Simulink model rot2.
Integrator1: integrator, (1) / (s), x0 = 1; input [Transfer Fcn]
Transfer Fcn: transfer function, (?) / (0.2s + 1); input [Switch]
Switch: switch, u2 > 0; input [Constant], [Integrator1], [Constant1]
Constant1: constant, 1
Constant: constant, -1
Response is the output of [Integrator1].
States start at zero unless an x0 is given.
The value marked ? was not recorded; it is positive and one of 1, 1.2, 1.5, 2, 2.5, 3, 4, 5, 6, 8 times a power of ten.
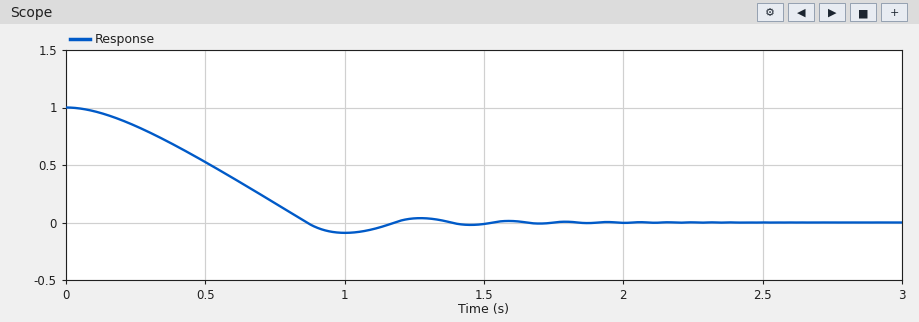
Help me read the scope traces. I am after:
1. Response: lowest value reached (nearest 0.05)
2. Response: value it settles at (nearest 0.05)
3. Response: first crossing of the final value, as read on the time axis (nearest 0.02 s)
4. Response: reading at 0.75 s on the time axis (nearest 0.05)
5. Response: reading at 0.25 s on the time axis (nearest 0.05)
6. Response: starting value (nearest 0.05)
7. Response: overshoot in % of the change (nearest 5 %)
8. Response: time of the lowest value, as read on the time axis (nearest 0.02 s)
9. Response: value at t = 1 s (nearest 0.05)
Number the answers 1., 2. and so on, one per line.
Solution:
1. -0.10
2. 0.00
3. 0.86 s
4. 0.15
5. 0.85
6. 1.00
7. 10 %
8. 1.00 s
9. -0.10
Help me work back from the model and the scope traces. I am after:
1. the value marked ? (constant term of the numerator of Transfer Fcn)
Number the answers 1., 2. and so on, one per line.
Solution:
1. 1.5
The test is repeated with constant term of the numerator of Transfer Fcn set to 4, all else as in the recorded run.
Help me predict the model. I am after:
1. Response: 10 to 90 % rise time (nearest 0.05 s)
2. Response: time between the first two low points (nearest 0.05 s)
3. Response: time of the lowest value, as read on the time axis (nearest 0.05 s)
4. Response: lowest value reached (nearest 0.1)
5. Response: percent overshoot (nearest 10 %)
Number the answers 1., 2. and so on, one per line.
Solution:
1. 0.30 s
2. 0.40 s
3. 0.55 s
4. -0.2
5. 20 %
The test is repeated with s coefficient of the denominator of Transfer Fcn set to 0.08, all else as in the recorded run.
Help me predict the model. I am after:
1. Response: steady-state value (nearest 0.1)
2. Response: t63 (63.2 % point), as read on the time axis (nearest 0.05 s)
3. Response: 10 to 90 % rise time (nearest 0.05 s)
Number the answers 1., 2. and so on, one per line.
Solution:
1. 0.0
2. 0.50 s
3. 0.55 s
